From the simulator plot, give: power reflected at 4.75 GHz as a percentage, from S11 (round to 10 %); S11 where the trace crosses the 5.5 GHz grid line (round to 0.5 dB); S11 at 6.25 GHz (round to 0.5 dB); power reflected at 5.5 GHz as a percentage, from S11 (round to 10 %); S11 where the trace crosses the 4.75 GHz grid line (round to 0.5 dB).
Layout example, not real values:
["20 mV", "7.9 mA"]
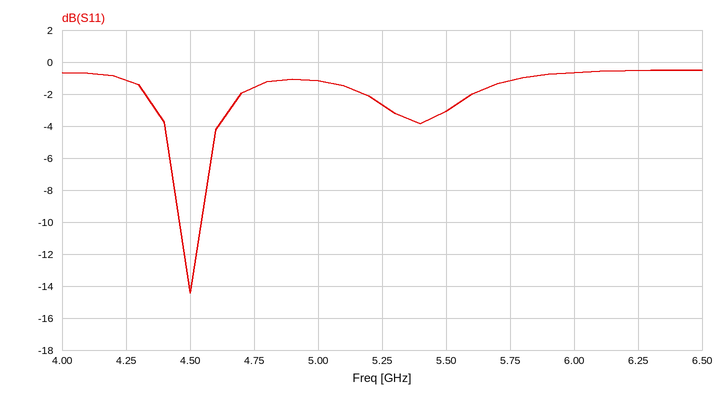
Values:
["70 %", "-3.0 dB", "-0.5 dB", "50 %", "-1.5 dB"]
